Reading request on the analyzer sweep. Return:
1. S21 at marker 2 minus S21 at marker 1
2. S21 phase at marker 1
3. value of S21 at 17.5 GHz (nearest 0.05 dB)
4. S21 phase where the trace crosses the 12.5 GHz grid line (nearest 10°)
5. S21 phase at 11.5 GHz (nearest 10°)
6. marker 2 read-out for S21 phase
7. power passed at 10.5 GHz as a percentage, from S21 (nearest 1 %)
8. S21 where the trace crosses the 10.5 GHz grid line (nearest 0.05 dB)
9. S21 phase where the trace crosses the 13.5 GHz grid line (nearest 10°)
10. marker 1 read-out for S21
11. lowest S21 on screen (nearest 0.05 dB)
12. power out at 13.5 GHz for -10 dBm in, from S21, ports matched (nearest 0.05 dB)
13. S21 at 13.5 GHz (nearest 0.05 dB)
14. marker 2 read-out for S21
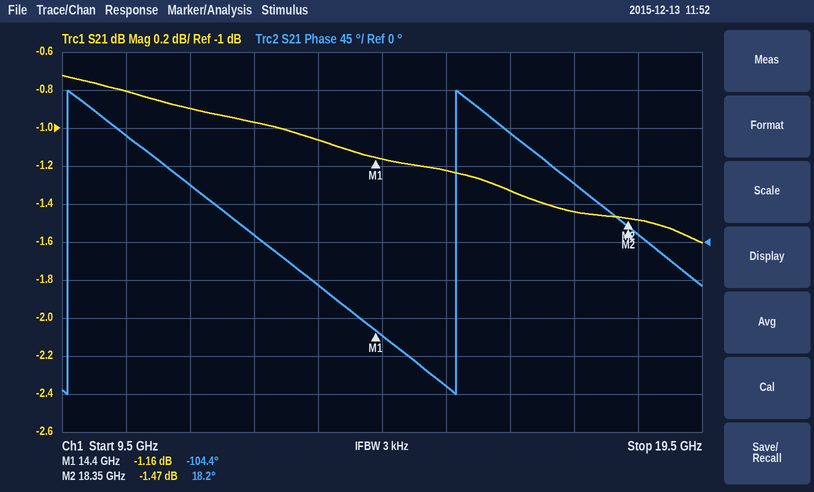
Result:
-0.31 dB
-104.4°
-1.45 dB
10°
70°
18.2°
83 %
-0.80 dB
-50°
-1.16 dB
-1.60 dB
-11.05 dBm
-1.05 dB
-1.47 dB
